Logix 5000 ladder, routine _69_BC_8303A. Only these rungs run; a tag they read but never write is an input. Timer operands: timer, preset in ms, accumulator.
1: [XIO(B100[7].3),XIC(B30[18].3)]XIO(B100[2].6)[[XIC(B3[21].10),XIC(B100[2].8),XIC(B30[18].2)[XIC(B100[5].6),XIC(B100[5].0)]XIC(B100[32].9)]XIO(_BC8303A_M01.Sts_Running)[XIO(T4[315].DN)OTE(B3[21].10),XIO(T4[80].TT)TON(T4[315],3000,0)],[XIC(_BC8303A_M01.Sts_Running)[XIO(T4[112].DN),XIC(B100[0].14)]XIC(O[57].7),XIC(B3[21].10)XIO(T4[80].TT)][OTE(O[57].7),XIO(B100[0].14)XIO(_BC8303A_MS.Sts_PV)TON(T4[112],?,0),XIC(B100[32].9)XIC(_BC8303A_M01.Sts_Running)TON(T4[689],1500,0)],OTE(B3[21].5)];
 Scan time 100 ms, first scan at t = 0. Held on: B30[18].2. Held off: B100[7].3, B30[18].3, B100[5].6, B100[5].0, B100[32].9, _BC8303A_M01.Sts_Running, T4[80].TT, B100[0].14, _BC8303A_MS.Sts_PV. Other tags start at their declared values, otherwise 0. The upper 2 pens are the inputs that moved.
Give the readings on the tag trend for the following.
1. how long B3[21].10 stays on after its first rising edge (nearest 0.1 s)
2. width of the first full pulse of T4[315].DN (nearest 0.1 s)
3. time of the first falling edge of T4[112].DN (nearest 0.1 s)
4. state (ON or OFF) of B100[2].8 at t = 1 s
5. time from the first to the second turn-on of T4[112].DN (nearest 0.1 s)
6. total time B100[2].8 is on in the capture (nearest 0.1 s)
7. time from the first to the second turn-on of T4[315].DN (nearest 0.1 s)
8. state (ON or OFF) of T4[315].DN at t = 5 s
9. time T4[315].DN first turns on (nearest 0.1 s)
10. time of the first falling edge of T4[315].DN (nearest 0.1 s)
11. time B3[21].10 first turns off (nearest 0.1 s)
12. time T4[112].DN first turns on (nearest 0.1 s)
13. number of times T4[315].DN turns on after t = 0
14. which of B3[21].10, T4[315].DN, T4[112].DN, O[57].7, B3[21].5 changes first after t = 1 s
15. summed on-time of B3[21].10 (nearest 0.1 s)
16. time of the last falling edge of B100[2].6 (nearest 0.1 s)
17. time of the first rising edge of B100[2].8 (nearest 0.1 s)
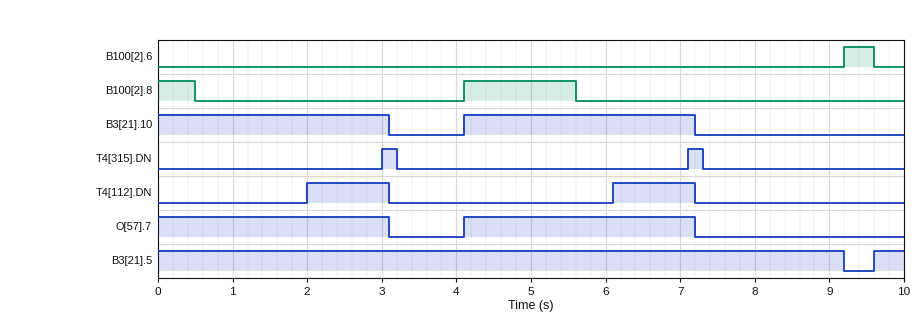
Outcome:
3.1 s
0.2 s
3.1 s
OFF
4.1 s
2.0 s
4.1 s
OFF
3.0 s
3.2 s
3.1 s
2.0 s
2
T4[112].DN
6.2 s
9.6 s
4.1 s
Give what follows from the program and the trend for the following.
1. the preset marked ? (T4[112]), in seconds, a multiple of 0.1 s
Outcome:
2.0 s
